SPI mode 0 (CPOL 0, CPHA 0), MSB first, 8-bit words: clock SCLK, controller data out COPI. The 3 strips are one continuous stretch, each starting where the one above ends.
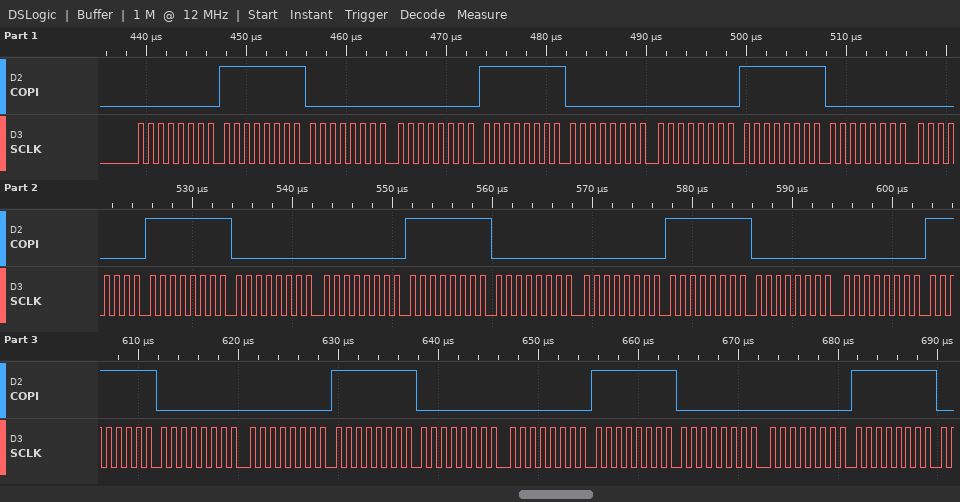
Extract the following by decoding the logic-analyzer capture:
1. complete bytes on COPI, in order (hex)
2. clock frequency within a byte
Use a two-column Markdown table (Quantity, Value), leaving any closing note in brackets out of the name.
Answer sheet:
| Quantity | Value |
|---|---|
| complete bytes on COPI, in order | 0x00 0xFF 0x00 0x00 0xFF 0x00 0x00 0xFF 0x00 0x00 0xFF 0x00 0x00 0xFF 0x00 0x00 0xFF 0x00 0x00 0xFF 0x00 0x00 0xFF 0x00 0x00 0xFF 0x00 0x00 0xFF |
| clock frequency within a byte | 1 MHz |
